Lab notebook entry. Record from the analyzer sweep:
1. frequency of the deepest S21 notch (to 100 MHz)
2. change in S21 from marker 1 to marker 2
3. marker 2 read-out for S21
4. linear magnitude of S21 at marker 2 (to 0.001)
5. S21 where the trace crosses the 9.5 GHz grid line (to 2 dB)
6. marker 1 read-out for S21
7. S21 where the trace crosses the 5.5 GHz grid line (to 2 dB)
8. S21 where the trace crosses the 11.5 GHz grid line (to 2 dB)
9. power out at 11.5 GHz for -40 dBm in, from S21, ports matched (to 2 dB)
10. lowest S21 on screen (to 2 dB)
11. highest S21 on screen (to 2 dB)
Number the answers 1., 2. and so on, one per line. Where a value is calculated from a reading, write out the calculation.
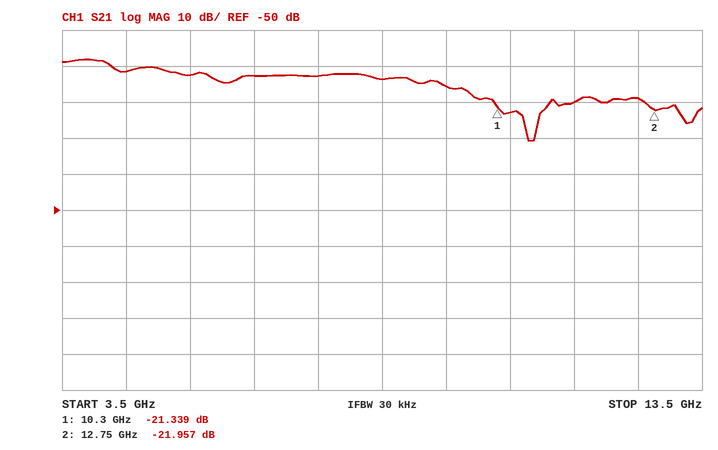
1. 10.8 GHz
2. -21.957 − (-21.339) = -0.618 dB
3. -21.957 dB
4. 10^(-21.957/20) ≈ 0.080
5. -16 dB
6. -21.339 dB
7. -12 dB
8. -20 dB
9. -40 dBm + (-20 dB) = -60 dBm
10. -30 dB
11. -8 dB
